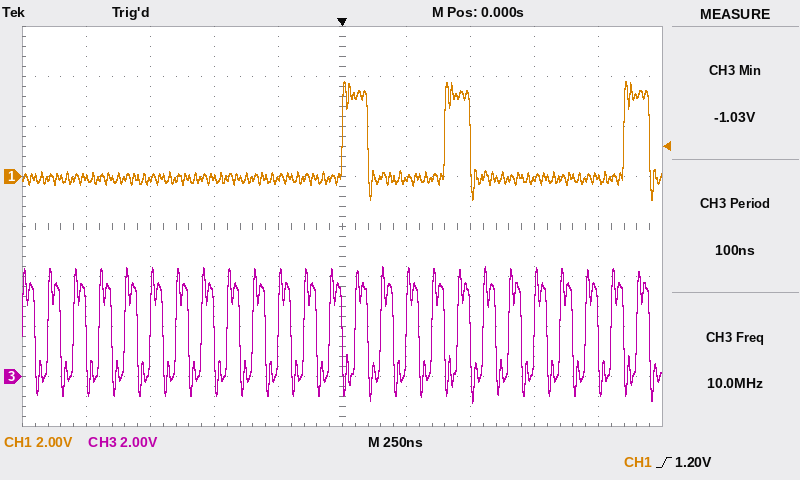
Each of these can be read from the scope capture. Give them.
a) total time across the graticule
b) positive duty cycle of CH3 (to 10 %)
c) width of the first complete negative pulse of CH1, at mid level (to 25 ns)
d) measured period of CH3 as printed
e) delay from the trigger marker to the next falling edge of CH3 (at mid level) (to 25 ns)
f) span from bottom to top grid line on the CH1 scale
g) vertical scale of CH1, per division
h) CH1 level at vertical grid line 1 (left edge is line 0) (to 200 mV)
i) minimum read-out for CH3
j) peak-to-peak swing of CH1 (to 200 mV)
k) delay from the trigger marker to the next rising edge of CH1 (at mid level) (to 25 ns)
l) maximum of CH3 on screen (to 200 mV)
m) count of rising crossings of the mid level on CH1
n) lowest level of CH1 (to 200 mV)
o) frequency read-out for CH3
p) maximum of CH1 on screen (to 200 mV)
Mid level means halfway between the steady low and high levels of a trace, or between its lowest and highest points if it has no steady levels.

2.5 µs
50 %
300 ns
100 ns
100 ns
16 V
2 V
0.0 V
-1.03 V
4.8 V
400 ns
4.4 V
3
-1.0 V
10.0 MHz
3.8 V
